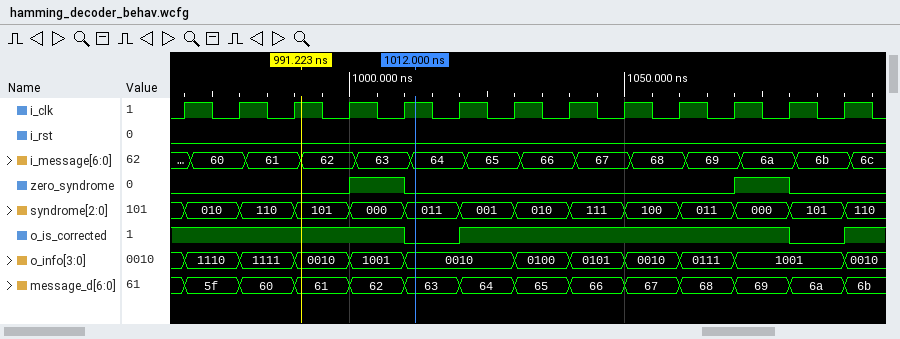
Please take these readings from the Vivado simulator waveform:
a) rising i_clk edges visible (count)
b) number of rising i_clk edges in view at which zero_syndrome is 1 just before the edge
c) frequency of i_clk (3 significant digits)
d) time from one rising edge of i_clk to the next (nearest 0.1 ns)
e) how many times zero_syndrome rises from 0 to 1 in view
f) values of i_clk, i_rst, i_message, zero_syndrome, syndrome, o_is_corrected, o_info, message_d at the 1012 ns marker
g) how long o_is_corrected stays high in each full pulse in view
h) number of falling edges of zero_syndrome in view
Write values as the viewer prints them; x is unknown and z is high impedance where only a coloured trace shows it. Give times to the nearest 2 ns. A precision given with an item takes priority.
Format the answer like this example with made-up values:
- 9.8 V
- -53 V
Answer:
- 13
- 2
- 100 MHz
- 10 ns
- 2
- i_clk=1, i_rst=0, i_message=64, zero_syndrome=0, syndrome=011, o_is_corrected=0, o_info=0010, message_d=63
- 60 ns
- 2
